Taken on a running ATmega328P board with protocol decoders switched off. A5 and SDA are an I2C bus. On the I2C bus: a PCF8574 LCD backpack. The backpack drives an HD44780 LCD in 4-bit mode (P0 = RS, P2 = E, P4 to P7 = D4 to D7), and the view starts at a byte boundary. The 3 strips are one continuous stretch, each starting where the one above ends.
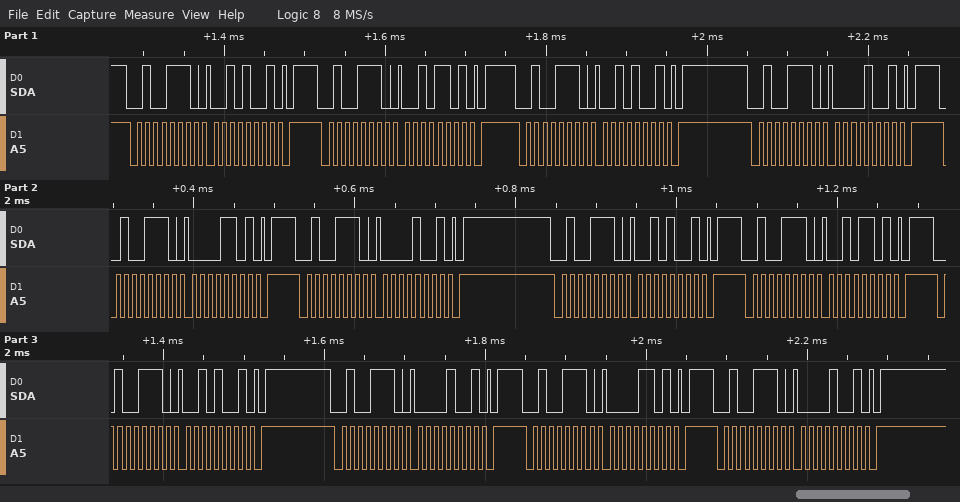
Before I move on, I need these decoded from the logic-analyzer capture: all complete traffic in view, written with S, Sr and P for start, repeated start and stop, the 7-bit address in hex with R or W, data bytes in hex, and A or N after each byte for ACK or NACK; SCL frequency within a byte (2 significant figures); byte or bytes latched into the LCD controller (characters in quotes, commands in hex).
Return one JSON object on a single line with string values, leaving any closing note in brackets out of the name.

{"all complete traffic in view, written with S, Sr and P for start, repeated start and stop, the 7-bit address in hex with R or W, data bytes in hex, and A or N after each byte for ACK or NACK": "S 27W A 29 A P S 27W A 2D A P S 27W A 29 A P S 27W A 09 A P S 27W A 0D A P S 27W A 09 A P S 27W A 29 A P S 27W A 2D A P S 27W A 29 A P S 27W A 09 A P S 27W A 0D A P S 27W A 09 A P", "SCL frequency within a byte": "100 kHz", "byte or bytes latched into the LCD controller": "' ' ' '"}
